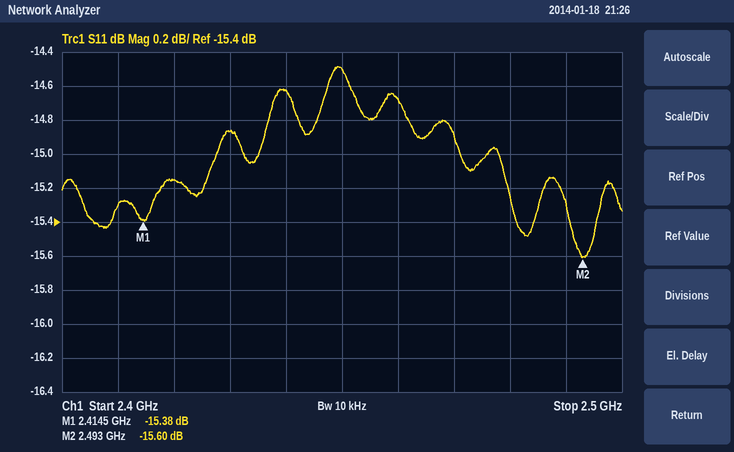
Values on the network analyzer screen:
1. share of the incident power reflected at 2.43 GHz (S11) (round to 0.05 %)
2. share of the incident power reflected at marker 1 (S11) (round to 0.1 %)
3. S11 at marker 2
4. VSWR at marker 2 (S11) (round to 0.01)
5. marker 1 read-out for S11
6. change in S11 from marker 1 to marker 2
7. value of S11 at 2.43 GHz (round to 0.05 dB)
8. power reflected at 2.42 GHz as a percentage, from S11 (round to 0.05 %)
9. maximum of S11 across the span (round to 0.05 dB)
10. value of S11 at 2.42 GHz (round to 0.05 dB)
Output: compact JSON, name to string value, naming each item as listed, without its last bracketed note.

{"share of the incident power reflected at 2.43 GHz (S11)": "3.25 %", "share of the incident power reflected at marker 1 (S11)": "2.9 %", "S11 at marker 2": "-15.60 dB", "VSWR at marker 2 (S11)": "1.40", "marker 1 read-out for S11": "-15.38 dB", "change in S11 from marker 1 to marker 2": "-0.22 dB", "value of S11 at 2.43 GHz": "-14.85 dB", "power reflected at 2.42 GHz as a percentage, from S11": "3.05 %", "maximum of S11 across the span": "-14.50 dB", "value of S11 at 2.42 GHz": "-15.15 dB"}
